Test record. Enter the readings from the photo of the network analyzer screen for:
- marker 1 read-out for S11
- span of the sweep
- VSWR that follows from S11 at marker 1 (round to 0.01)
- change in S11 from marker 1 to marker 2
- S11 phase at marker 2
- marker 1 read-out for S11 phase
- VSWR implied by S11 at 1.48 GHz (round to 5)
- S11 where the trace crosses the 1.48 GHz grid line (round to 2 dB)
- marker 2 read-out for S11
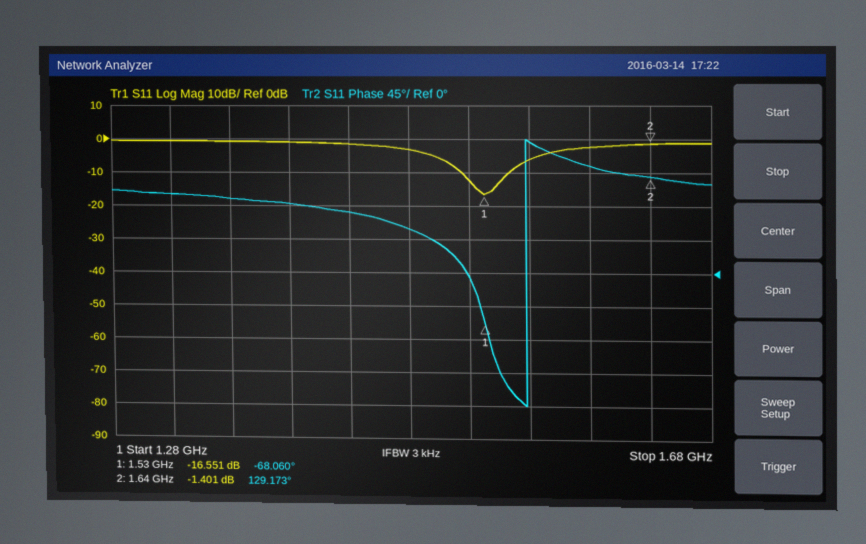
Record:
-16.551 dB
400 MHz
1.35
15.150 dB
129.173°
-68.060°
5
-4 dB
-1.401 dB
